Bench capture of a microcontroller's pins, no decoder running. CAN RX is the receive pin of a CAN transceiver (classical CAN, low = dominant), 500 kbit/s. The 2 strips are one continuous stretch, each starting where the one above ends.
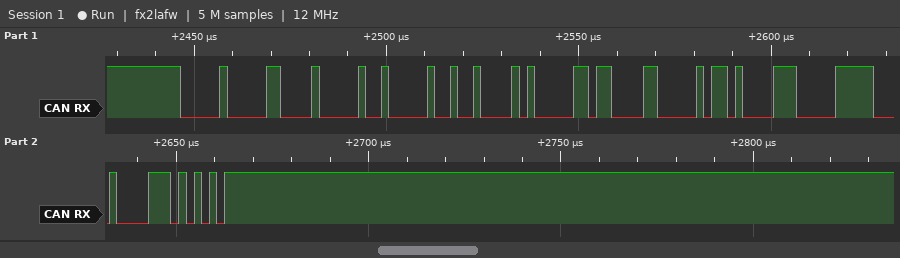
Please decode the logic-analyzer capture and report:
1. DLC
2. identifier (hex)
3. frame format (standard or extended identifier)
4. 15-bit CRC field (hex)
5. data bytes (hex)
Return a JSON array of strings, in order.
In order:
["8", "0x002", "standard", "0x10EA", "08 09 0A 0B 0C 0D 0E 0F"]
